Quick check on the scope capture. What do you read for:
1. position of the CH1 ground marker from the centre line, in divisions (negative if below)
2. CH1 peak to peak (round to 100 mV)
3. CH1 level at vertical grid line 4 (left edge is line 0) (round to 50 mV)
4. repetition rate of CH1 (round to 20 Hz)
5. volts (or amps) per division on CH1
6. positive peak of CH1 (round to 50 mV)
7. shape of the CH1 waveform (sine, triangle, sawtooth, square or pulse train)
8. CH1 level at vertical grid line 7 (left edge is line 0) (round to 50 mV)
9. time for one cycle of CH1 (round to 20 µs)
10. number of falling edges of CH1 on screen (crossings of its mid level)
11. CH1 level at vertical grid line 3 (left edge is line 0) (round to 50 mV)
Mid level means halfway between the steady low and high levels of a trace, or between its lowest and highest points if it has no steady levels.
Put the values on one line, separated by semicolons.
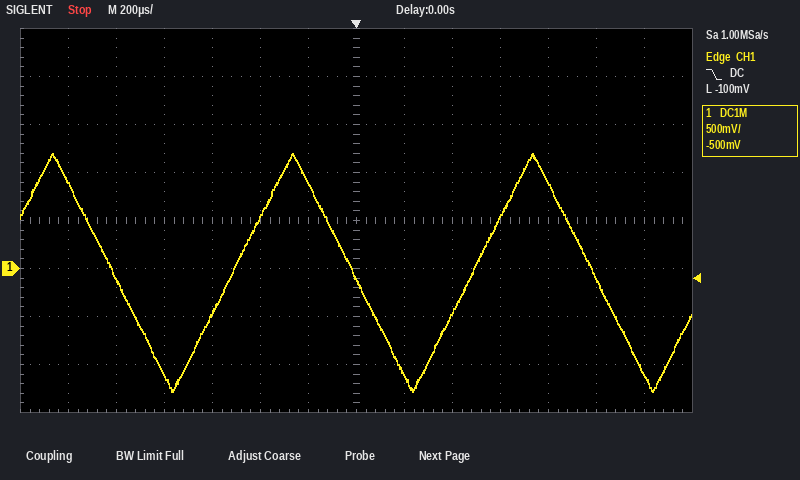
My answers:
-1.0 div; 2.50 V; -450 mV; 1.00 kHz; 500 mV; 1.20 V; triangle; -100 mV; 1.00 ms; 3; -1.10 V
